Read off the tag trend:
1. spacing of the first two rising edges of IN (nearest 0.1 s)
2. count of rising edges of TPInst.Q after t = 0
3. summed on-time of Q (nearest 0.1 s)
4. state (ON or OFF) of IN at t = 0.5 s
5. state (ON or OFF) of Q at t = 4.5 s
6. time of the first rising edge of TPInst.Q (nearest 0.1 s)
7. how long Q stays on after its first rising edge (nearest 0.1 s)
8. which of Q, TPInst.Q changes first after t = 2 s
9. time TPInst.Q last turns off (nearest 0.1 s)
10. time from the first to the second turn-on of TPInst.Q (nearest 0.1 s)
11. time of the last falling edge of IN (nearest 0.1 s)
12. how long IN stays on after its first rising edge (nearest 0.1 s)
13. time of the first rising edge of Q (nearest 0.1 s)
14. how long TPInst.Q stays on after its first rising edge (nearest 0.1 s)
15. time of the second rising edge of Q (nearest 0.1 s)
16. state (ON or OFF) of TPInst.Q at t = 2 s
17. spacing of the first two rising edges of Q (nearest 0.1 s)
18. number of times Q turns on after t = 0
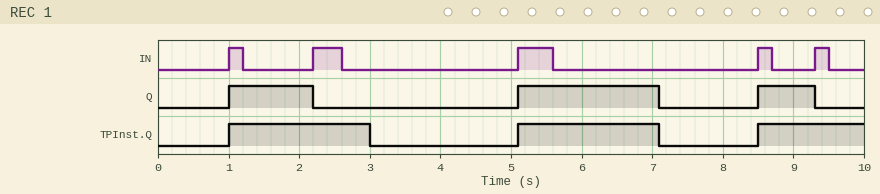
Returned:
1.2 s
3
4.0 s
OFF
OFF
1.0 s
1.2 s
Q
7.1 s
4.1 s
9.5 s
0.2 s
1.0 s
2.0 s
5.1 s
ON
4.1 s
3
